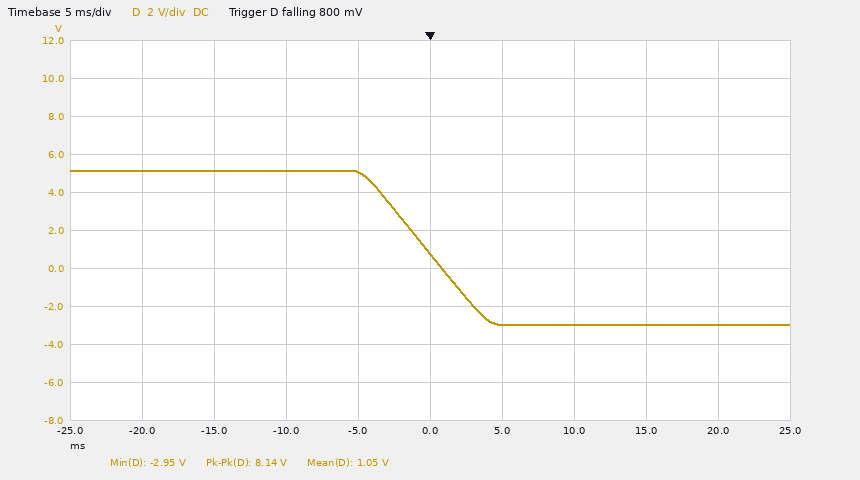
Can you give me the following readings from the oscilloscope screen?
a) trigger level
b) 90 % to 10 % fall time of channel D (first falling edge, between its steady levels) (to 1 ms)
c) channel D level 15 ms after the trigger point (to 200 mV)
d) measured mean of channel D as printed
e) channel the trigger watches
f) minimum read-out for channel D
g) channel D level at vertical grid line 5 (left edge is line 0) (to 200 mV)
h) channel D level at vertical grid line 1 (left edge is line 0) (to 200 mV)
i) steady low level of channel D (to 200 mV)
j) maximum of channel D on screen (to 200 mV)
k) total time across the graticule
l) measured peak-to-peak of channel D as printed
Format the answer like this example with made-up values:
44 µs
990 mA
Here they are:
800 mV
7 ms
-3.0 V
1.05 V
channel D
-2.95 V
800 mV
5.2 V
-3.0 V
5.2 V
50 ms
8.14 V
